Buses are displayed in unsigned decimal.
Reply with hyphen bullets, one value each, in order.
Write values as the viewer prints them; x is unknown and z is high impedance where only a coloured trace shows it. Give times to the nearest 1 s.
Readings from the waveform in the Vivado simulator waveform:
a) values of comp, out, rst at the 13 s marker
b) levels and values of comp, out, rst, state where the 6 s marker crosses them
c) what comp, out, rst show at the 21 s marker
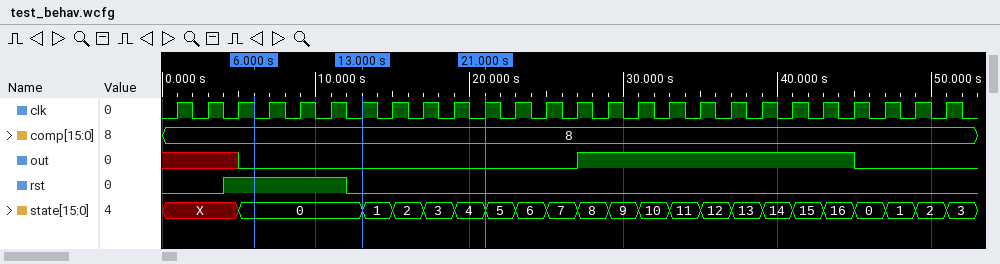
- comp=8, out=0, rst=0
- comp=8, out=0, rst=1, state=0
- comp=8, out=0, rst=0
